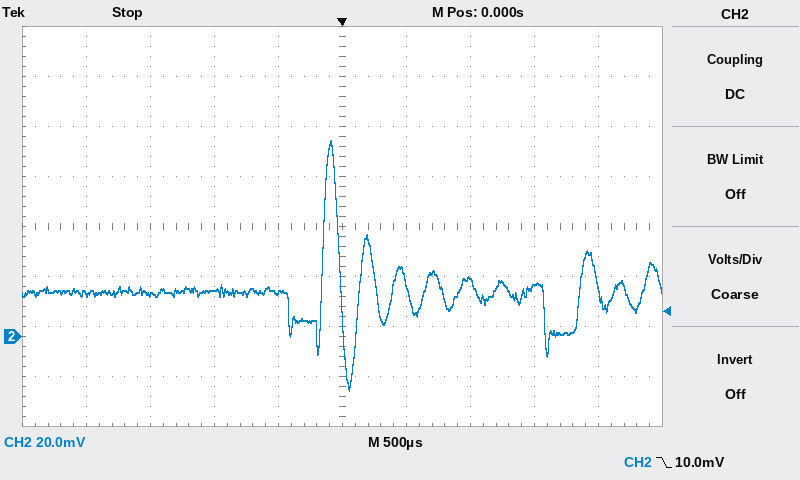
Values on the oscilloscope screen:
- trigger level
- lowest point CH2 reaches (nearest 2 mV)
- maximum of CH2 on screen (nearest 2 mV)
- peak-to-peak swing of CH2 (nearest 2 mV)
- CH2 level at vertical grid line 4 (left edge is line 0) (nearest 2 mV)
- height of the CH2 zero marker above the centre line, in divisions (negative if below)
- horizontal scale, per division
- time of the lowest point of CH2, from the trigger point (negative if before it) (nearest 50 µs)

10.0 mV
-22 mV
78 mV
100 mV
18 mV
-2.2 div
500 µs
+50 µs
